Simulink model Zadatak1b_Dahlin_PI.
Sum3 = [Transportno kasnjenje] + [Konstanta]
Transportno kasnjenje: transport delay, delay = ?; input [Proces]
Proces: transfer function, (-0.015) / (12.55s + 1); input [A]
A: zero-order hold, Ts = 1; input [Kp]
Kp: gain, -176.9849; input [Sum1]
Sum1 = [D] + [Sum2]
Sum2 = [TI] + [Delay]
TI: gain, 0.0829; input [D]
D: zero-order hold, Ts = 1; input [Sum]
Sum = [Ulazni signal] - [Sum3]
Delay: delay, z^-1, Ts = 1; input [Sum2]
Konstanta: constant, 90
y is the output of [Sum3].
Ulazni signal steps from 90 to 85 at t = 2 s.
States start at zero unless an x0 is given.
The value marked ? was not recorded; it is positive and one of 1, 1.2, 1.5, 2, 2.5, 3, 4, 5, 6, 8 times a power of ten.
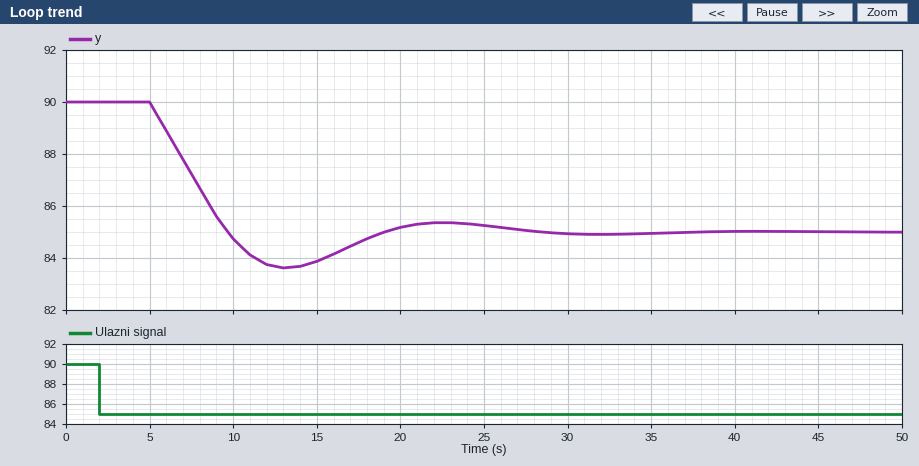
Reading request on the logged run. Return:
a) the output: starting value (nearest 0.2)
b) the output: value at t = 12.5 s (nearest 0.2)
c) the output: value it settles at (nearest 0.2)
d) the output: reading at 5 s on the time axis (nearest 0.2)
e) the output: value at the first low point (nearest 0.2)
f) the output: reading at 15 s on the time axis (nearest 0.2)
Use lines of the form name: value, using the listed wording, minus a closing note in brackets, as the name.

the output: starting value: 90.0
the output: value at t = 12.5 s: 83.6
the output: value it settles at: 85.0
the output: reading at 5 s on the time axis: 90.0
the output: value at the first low point: 83.6
the output: reading at 15 s on the time axis: 83.8
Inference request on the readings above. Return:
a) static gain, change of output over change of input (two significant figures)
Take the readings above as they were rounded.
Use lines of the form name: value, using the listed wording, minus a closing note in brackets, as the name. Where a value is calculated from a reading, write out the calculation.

static gain, change of output over change of input: (85 - 90) / (85 - 90) = 1.0
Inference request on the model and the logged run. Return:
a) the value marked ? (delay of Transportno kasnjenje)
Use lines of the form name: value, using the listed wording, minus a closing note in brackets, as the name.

the value marked ?: 3
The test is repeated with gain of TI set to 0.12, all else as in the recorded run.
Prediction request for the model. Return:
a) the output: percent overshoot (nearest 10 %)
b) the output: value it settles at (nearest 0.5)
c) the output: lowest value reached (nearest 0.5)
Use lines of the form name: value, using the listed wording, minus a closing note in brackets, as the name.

the output: percent overshoot: 40 %
the output: value it settles at: 85.0
the output: lowest value reached: 83.0
